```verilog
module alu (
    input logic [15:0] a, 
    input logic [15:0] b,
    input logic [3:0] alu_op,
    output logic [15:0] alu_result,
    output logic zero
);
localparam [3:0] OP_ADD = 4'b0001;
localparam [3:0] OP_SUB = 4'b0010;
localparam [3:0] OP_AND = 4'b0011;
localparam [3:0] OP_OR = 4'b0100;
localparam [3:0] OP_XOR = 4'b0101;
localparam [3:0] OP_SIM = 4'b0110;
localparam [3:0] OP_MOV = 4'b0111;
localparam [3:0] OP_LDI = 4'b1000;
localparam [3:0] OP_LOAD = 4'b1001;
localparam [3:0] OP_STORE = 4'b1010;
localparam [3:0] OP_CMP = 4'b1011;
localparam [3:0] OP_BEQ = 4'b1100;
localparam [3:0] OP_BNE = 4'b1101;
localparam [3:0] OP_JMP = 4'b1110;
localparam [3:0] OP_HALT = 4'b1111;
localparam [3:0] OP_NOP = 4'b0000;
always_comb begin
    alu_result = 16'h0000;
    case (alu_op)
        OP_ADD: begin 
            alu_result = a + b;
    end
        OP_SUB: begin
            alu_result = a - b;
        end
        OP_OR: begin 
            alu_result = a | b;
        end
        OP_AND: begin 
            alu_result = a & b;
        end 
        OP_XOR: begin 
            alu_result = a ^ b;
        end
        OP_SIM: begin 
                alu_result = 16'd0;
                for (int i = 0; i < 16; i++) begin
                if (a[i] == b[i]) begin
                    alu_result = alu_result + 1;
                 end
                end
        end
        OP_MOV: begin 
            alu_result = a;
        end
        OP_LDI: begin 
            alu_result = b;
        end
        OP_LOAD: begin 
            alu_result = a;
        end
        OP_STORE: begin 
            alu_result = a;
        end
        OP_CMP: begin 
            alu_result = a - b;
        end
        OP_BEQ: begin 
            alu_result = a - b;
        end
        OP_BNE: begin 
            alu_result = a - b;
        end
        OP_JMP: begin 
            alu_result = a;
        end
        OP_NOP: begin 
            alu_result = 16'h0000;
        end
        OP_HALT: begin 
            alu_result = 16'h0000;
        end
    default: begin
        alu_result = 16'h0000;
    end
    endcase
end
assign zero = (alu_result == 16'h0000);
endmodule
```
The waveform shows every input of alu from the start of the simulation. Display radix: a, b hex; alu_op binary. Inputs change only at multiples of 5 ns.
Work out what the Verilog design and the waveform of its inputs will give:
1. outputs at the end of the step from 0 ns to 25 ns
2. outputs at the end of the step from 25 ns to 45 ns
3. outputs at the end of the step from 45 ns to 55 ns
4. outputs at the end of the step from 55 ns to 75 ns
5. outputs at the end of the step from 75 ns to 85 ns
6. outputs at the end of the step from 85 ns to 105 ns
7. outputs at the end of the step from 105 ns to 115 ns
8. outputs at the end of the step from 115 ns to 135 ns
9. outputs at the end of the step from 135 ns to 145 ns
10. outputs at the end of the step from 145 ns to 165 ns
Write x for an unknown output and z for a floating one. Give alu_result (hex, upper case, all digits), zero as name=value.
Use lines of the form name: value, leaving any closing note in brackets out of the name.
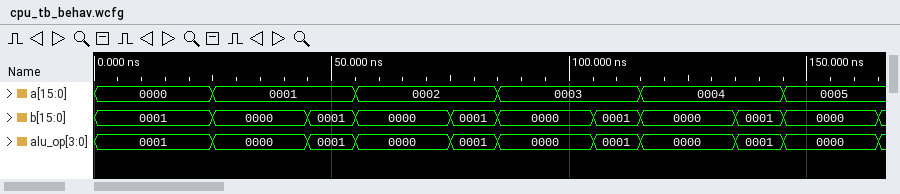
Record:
outputs at the end of the step from 0 ns to 25 ns: alu_result=0001, zero=0
outputs at the end of the step from 25 ns to 45 ns: alu_result=0000, zero=1
outputs at the end of the step from 45 ns to 55 ns: alu_result=0002, zero=0
outputs at the end of the step from 55 ns to 75 ns: alu_result=0000, zero=1
outputs at the end of the step from 75 ns to 85 ns: alu_result=0003, zero=0
outputs at the end of the step from 85 ns to 105 ns: alu_result=0000, zero=1
outputs at the end of the step from 105 ns to 115 ns: alu_result=0004, zero=0
outputs at the end of the step from 115 ns to 135 ns: alu_result=0000, zero=1
outputs at the end of the step from 135 ns to 145 ns: alu_result=0005, zero=0
outputs at the end of the step from 145 ns to 165 ns: alu_result=0000, zero=1
